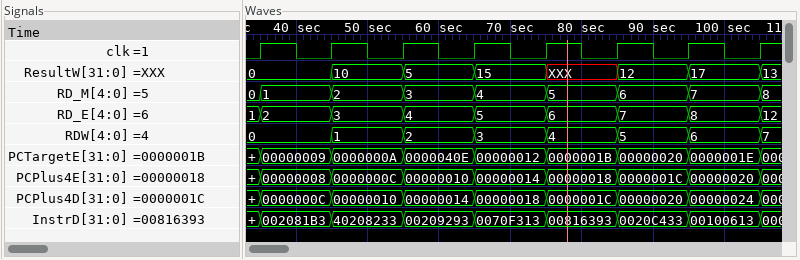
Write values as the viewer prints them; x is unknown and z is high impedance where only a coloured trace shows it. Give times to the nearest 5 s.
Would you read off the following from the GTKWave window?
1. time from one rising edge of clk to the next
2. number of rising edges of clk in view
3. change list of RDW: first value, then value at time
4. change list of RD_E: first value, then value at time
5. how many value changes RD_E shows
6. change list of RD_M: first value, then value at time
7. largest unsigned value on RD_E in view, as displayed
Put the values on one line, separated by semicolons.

10 s; 8; 0, 1 at 45 s, 2 at 55 s, 3 at 65 s, 4 at 75 s, 5 at 85 s, 6 at 95 s, 7 at 105 s; 1, 2 at 35 s, 3 at 45 s, 4 at 55 s, 5 at 65 s, 6 at 75 s, 7 at 85 s, 8 at 95 s, 12 at 105 s; 8; 0, 1 at 35 s, 2 at 45 s, 3 at 55 s, 4 at 65 s, 5 at 75 s, 6 at 85 s, 7 at 95 s, 8 at 105 s; 12
